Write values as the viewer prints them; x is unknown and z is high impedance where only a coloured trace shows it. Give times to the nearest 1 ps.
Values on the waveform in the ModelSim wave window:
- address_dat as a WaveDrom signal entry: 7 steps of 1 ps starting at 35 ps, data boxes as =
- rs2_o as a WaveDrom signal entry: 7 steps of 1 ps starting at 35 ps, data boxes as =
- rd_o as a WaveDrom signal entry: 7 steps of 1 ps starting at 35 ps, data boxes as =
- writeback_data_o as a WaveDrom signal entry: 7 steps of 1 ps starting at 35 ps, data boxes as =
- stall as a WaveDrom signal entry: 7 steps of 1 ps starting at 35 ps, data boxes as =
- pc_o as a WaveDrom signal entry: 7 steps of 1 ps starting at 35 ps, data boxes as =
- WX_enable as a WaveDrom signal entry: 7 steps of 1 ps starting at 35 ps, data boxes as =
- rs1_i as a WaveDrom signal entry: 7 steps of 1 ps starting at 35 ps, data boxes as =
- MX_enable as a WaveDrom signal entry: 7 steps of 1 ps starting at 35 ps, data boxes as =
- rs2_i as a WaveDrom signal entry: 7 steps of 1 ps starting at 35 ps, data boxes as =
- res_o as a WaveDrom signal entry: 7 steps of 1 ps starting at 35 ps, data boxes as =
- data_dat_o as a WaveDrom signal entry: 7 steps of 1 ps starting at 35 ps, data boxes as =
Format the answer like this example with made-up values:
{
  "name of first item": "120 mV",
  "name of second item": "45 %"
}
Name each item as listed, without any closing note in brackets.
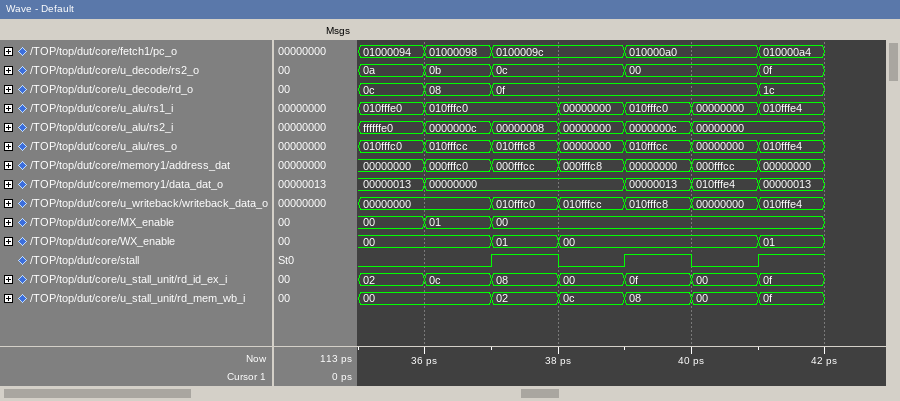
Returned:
{
  "address_dat as a WaveDrom signal entry: 7 steps of 1 ps starting at 35 ps, data boxes as =": "{name: 'address_dat', wave: '=======', data: '00000000 000fffc0 000fffcc 000fffc8 00000000 000fffcc 00000000'}",
  "rs2_o as a WaveDrom signal entry: 7 steps of 1 ps starting at 35 ps, data boxes as =": "{name: 'rs2_o', wave: '===.=.=', data: '0a 0b 0c 00 0f'}",
  "rd_o as a WaveDrom signal entry: 7 steps of 1 ps starting at 35 ps, data boxes as =": "{name: 'rd_o', wave: '===...=', data: '0c 08 0f 1c'}",
  "writeback_data_o as a WaveDrom signal entry: 7 steps of 1 ps starting at 35 ps, data boxes as =": "{name: 'writeback_data_o', wave: '=.=====', data: '00000000 010fffc0 010fffcc 010fffc8 00000000 010fffe4'}",
  "stall as a WaveDrom signal entry: 7 steps of 1 ps starting at 35 ps, data boxes as =": "{name: 'stall', wave: '0.10101'}",
  "pc_o as a WaveDrom signal entry: 7 steps of 1 ps starting at 35 ps, data boxes as =": "{name: 'pc_o', wave: '===.=.=', data: '01000094 01000098 0100009c 010000a0 010000a4'}",
  "WX_enable as a WaveDrom signal entry: 7 steps of 1 ps starting at 35 ps, data boxes as =": "{name: 'WX_enable', wave: '=.==..=', data: '00 01 00 01'}",
  "rs1_i as a WaveDrom signal entry: 7 steps of 1 ps starting at 35 ps, data boxes as =": "{name: 'rs1_i', wave: '==.====', data: '010fffe0 010fffc0 00000000 010fffc0 00000000 010fffe4'}",
  "MX_enable as a WaveDrom signal entry: 7 steps of 1 ps starting at 35 ps, data boxes as =": "{name: 'MX_enable', wave: '===....', data: '00 01 00'}",
  "rs2_i as a WaveDrom signal entry: 7 steps of 1 ps starting at 35 ps, data boxes as =": "{name: 'rs2_i', wave: '======.', data: 'ffffffe0 0000000c 00000008 00000000 0000000c 00000000'}",
  "res_o as a WaveDrom signal entry: 7 steps of 1 ps starting at 35 ps, data boxes as =": "{name: 'res_o', wave: '=======', data: '010fffc0 010fffcc 010fffc8 00000000 010fffcc 00000000 010fffe4'}",
  "data_dat_o as a WaveDrom signal entry: 7 steps of 1 ps starting at 35 ps, data boxes as =": "{name: 'data_dat_o', wave: '==..===', data: '00000013 00000000 00000013 010fffe4 00000013'}"
}
